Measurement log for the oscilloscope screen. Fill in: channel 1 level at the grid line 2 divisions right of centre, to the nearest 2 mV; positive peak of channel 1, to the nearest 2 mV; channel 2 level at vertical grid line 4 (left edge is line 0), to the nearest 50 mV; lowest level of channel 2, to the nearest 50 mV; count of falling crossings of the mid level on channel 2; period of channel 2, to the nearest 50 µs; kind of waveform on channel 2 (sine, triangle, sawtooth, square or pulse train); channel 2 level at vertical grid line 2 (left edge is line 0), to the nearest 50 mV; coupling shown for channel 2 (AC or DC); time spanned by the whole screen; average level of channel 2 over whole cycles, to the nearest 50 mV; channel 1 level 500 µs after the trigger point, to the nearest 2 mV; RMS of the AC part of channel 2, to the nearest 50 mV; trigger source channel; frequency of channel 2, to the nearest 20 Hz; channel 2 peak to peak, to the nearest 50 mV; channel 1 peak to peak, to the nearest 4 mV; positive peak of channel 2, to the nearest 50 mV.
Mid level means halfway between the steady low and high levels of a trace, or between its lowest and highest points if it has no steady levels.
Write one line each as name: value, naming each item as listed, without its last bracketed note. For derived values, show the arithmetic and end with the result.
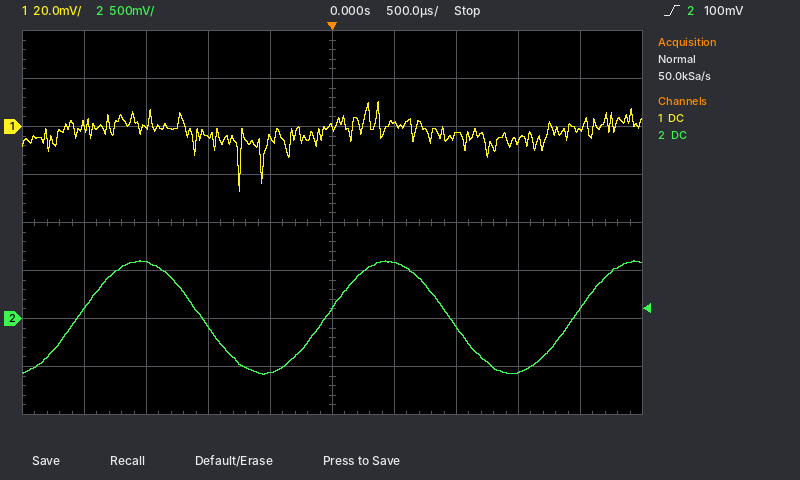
channel 1 level at the grid line 2 divisions right of centre, to the nearest 2 mV: -4 mV
positive peak of channel 1, to the nearest 2 mV: 10 mV
channel 2 level at vertical grid line 4 (left edge is line 0), to the nearest 50 mV: -550 mV
lowest level of channel 2, to the nearest 50 mV: -600 mV
count of falling crossings of the mid level on channel 2: 2
period of channel 2, to the nearest 50 µs: 2.00 ms
kind of waveform on channel 2: sine
channel 2 level at vertical grid line 2 (left edge is line 0), to the nearest 50 mV: 600 mV
coupling shown for channel 2: DC
time spanned by the whole screen: 5 ms
average level of channel 2 over whole cycles, to the nearest 50 mV: (600 mV + (-600 mV)) / 2 ≈ 0 mV
channel 1 level 500 µs after the trigger point, to the nearest 2 mV: 2 mV
RMS of the AC part of channel 2, to the nearest 50 mV: 1.20 V / (2√2) ≈ 424 mV, so 400 mV to the nearest 50 mV
trigger source channel: channel 2
frequency of channel 2, to the nearest 20 Hz: 1 / 2.00 ms ≈ 500 Hz
channel 2 peak to peak, to the nearest 50 mV: 600 mV − (-600 mV) = 1.20 V
channel 1 peak to peak, to the nearest 4 mV: 36 mV
positive peak of channel 2, to the nearest 50 mV: 600 mV
